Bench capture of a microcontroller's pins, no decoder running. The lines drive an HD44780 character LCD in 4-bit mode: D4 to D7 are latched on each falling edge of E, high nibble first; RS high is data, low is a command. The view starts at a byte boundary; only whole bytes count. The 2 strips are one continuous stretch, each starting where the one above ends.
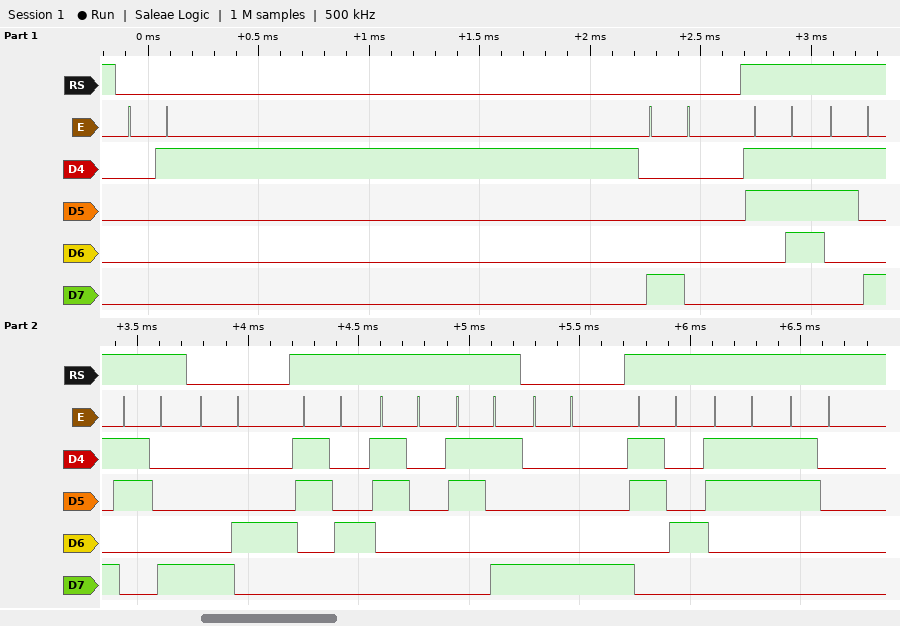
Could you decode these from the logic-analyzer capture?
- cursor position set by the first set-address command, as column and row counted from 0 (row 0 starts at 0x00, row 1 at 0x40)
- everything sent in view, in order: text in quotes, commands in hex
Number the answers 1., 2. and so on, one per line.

1. column 0, row 0
2. 0x01 0x80 "798" 0x84 "409" 0x88 "430"
